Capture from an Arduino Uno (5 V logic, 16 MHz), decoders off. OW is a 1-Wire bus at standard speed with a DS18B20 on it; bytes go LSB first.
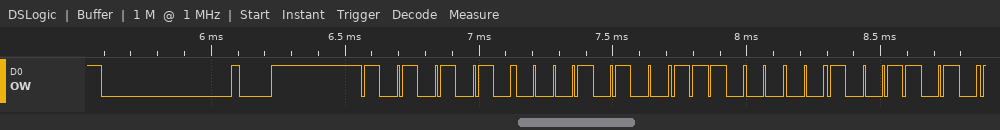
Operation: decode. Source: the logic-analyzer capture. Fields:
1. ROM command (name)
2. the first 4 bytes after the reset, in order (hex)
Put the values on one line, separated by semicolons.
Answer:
Match ROM; 55 28 07 59
